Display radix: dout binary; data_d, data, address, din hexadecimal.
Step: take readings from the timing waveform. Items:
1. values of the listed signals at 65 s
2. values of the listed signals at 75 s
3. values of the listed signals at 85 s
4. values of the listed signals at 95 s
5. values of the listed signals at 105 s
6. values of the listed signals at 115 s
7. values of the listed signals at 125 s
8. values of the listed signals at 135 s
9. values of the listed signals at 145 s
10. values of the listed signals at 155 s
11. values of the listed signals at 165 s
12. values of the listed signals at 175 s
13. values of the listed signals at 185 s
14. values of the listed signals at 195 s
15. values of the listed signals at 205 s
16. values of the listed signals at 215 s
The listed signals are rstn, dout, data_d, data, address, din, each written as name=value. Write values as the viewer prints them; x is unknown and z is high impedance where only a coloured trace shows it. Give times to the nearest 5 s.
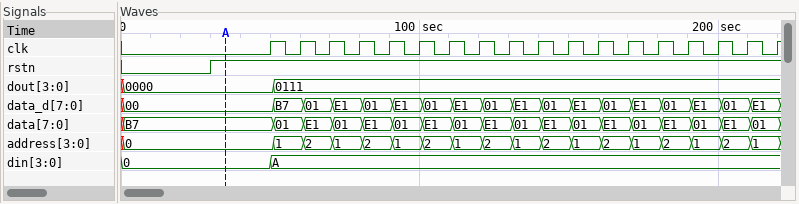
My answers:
rstn=1, dout=0111, data_d=01, data=E1, address=2, din=A
rstn=1, dout=0111, data_d=E1, data=01, address=1, din=A
rstn=1, dout=0111, data_d=01, data=E1, address=2, din=A
rstn=1, dout=0111, data_d=E1, data=01, address=1, din=A
rstn=1, dout=0111, data_d=01, data=E1, address=2, din=A
rstn=1, dout=0111, data_d=E1, data=01, address=1, din=A
rstn=1, dout=0111, data_d=01, data=E1, address=2, din=A
rstn=1, dout=0111, data_d=E1, data=01, address=1, din=A
rstn=1, dout=0111, data_d=01, data=E1, address=2, din=A
rstn=1, dout=0111, data_d=E1, data=01, address=1, din=A
rstn=1, dout=0111, data_d=01, data=E1, address=2, din=A
rstn=1, dout=0111, data_d=E1, data=01, address=1, din=A
rstn=1, dout=0111, data_d=01, data=E1, address=2, din=A
rstn=1, dout=0111, data_d=E1, data=01, address=1, din=A
rstn=1, dout=0111, data_d=01, data=E1, address=2, din=A
rstn=1, dout=0111, data_d=E1, data=01, address=1, din=A
